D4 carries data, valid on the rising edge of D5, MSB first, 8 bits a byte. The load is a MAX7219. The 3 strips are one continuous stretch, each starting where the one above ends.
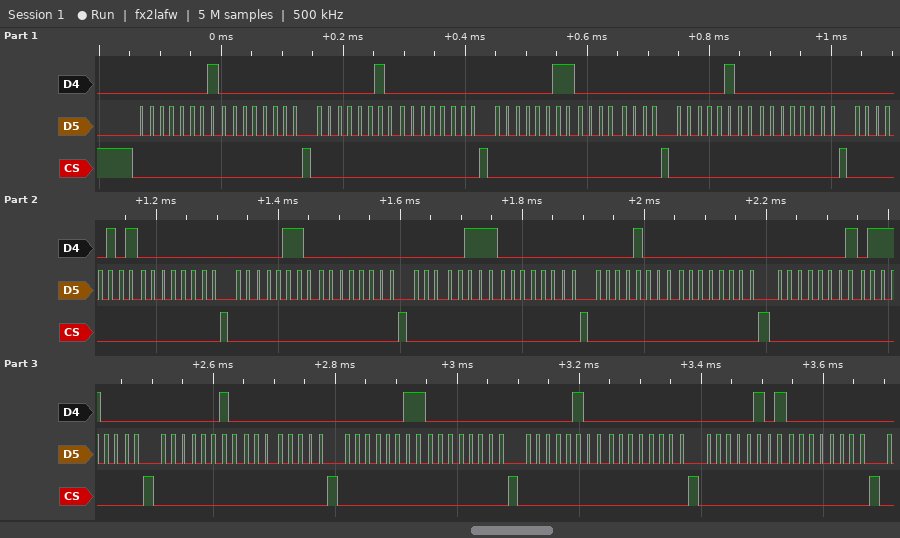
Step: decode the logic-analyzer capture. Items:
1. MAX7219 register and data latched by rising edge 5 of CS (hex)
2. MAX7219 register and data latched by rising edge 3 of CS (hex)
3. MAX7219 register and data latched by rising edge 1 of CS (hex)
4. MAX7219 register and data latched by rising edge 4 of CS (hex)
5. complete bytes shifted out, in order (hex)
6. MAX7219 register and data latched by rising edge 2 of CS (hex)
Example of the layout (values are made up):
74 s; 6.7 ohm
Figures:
register 0x5, data 0x00; register 0x3, data 0x00; register 0x1, data 0x00; register 0x4, data 0x00; 0x01 0x00 0x02 0x00 0x03 0x00 0x04 0x00 0x05 0x00 0x06 0x00 0x07 0x00 0x08 0x00 0x01 0x70 0x02 0x00 0x03 0x00 0x04 0x00 0x05 0x00; register 0x2, data 0x00
